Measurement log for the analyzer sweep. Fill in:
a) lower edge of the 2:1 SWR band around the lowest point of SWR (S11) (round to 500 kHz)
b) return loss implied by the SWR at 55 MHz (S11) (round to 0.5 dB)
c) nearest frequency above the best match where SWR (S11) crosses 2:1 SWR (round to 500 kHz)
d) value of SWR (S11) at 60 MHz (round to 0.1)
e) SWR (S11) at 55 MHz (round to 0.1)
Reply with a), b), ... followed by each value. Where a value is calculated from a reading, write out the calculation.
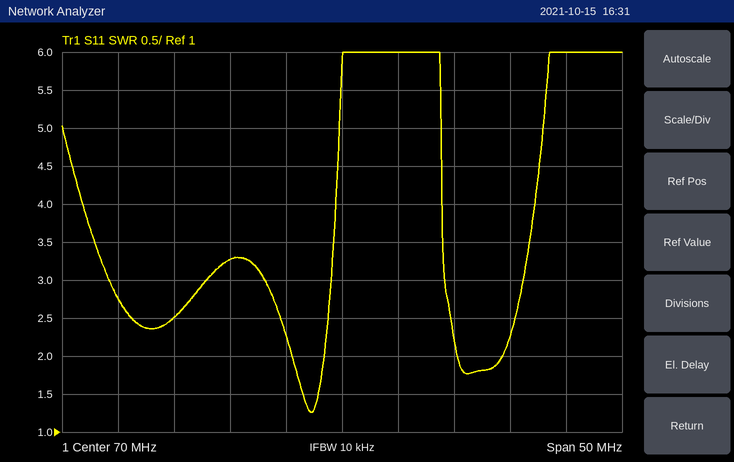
a) 65.5 MHz
b) −20 log10((2.5 − 1)/(2.5 + 1)) ≈ 7.36 dB, so 7.5 dB to the nearest 0.5 dB
c) 68.5 MHz
d) 3.3
e) 2.5
